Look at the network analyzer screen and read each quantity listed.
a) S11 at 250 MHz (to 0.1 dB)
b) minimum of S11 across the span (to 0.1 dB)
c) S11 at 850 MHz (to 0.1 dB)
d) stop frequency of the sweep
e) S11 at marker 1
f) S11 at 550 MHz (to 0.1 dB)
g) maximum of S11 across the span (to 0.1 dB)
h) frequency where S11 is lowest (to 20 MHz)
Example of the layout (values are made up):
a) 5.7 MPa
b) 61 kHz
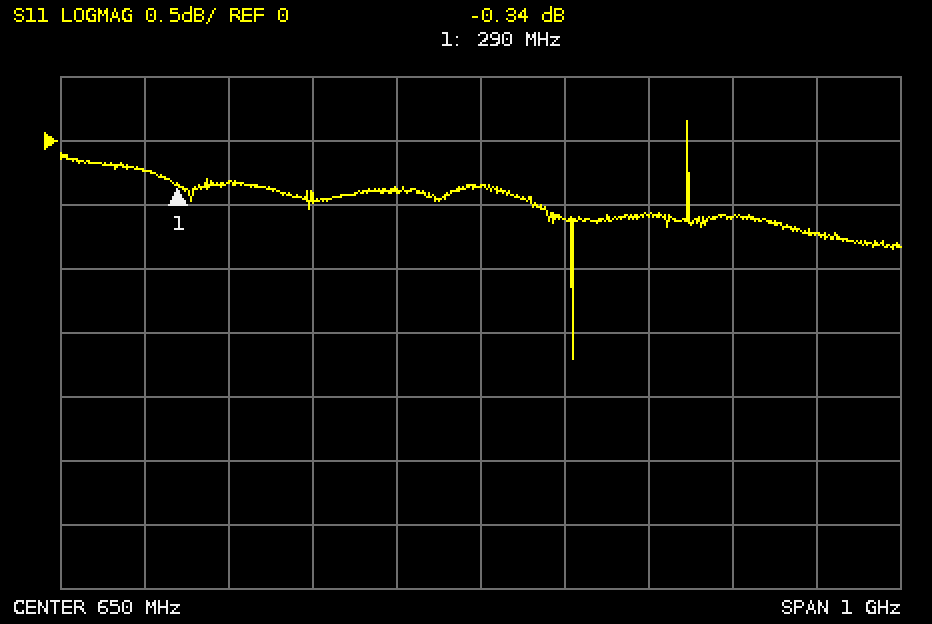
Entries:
a) -0.2 dB
b) -1.7 dB
c) -0.6 dB
d) 1.15 GHz
e) -0.34 dB
f) -0.4 dB
g) 0.2 dB
h) 760 MHz
